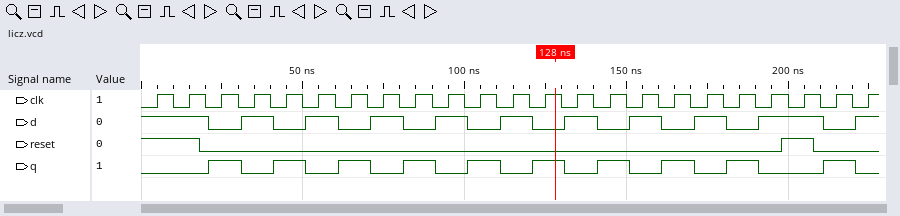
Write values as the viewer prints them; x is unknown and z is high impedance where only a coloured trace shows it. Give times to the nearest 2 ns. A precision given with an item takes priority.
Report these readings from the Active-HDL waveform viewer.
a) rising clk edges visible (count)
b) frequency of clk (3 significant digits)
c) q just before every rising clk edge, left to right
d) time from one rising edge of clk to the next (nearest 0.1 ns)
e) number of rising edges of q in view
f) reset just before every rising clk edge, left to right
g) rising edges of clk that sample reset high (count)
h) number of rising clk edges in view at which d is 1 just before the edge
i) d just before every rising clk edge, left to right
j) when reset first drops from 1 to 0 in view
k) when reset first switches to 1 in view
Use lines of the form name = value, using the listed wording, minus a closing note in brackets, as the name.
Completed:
rising clk edges visible = 23
frequency of clk = 100 MHz
q just before every rising clk edge, left to right = 0 0 1 0 1 0 1 0 1 0 1 0 1 0 1 0 1 0 1 0 0 1 0
time from one rising edge of clk to the next = 10 ns
number of rising edges of q in view = 10
reset just before every rising clk edge, left to right = 1 1 0 0 0 0 0 0 0 0 0 0 0 0 0 0 0 0 0 0 1 0 0
rising edges of clk that sample reset high = 3
number of rising clk edges in view at which d is 1 just before the edge = 13
d just before every rising clk edge, left to right = 1 1 0 1 0 1 0 1 0 1 0 1 0 1 0 1 0 1 0 1 1 0 1
when reset first drops from 1 to 0 in view = 18 ns
when reset first switches to 1 in view = 198 ns
